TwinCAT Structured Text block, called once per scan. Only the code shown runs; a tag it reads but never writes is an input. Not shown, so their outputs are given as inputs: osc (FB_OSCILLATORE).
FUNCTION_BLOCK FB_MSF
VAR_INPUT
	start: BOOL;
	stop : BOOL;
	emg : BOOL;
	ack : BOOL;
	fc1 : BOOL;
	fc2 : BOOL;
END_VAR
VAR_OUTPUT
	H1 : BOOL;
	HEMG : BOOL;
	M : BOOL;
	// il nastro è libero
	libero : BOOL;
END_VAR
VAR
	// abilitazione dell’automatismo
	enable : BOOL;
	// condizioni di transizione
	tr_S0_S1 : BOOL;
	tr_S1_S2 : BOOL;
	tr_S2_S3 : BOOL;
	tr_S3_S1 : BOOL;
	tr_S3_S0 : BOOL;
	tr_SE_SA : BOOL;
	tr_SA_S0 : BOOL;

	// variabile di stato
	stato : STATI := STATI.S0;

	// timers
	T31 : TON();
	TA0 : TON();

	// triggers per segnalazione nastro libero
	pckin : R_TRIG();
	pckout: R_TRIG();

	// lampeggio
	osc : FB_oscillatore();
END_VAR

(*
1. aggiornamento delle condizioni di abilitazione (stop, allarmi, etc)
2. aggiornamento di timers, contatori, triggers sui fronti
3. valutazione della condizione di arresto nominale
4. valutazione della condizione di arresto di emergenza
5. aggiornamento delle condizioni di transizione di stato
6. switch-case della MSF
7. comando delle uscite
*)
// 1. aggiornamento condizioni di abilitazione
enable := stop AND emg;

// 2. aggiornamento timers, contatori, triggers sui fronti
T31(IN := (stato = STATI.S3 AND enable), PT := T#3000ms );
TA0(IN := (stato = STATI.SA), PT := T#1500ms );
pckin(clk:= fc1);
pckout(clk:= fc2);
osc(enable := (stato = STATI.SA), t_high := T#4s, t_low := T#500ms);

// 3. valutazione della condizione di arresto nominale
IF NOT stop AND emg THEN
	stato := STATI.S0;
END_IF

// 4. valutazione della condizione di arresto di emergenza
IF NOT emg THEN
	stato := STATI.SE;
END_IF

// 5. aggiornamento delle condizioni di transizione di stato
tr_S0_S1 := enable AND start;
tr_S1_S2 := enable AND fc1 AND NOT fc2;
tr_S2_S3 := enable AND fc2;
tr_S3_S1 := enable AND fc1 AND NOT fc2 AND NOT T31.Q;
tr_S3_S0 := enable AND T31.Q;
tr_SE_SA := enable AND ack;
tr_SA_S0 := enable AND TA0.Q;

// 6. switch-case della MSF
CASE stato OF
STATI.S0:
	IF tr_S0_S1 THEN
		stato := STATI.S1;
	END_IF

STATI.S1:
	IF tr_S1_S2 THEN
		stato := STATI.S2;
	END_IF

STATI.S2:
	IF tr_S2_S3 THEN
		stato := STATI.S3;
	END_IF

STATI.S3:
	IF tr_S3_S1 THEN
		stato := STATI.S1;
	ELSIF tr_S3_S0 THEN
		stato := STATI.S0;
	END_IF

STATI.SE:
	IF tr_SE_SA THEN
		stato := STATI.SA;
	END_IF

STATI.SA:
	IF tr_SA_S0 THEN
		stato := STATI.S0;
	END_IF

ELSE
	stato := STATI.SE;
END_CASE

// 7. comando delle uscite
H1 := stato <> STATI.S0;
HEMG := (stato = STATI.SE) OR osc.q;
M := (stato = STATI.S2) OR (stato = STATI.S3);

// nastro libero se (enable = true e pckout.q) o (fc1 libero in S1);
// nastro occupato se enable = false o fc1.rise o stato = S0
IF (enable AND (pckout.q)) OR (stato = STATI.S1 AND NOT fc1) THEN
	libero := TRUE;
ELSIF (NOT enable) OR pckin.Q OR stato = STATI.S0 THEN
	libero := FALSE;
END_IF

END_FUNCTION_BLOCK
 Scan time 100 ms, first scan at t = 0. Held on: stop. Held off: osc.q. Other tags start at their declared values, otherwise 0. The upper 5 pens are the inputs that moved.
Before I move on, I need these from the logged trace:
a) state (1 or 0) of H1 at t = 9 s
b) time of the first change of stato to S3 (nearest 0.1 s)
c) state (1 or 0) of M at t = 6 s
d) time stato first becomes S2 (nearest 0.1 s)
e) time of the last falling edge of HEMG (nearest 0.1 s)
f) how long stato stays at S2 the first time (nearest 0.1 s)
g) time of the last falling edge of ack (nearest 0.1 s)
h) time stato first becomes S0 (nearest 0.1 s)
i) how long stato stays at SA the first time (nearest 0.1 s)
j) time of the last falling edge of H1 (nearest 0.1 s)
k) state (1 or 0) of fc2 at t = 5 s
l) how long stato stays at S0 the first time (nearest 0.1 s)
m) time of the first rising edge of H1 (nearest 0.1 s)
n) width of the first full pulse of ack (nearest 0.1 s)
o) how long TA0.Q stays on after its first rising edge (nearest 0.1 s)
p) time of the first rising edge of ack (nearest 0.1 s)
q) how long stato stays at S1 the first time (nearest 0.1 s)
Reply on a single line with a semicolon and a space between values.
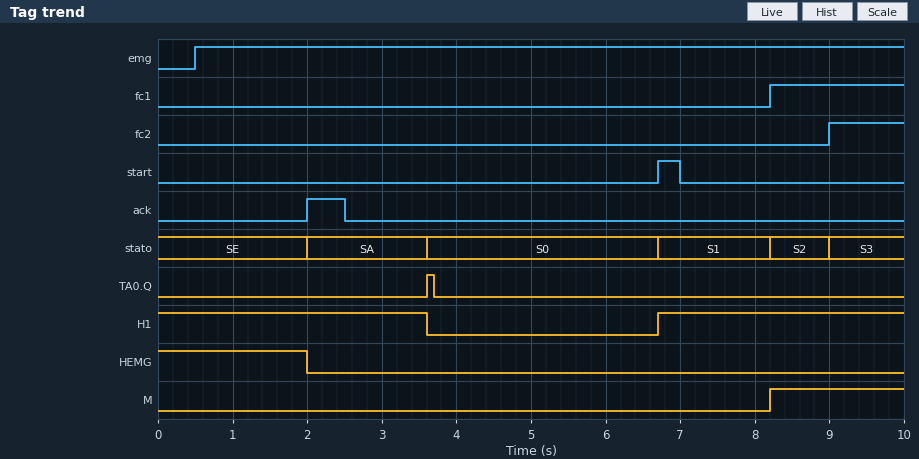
1; 9.0 s; 0; 8.2 s; 2.0 s; 0.8 s; 2.5 s; 3.6 s; 1.6 s; 3.6 s; 0; 3.1 s; 6.7 s; 0.5 s; 0.1 s; 2.0 s; 1.5 s
